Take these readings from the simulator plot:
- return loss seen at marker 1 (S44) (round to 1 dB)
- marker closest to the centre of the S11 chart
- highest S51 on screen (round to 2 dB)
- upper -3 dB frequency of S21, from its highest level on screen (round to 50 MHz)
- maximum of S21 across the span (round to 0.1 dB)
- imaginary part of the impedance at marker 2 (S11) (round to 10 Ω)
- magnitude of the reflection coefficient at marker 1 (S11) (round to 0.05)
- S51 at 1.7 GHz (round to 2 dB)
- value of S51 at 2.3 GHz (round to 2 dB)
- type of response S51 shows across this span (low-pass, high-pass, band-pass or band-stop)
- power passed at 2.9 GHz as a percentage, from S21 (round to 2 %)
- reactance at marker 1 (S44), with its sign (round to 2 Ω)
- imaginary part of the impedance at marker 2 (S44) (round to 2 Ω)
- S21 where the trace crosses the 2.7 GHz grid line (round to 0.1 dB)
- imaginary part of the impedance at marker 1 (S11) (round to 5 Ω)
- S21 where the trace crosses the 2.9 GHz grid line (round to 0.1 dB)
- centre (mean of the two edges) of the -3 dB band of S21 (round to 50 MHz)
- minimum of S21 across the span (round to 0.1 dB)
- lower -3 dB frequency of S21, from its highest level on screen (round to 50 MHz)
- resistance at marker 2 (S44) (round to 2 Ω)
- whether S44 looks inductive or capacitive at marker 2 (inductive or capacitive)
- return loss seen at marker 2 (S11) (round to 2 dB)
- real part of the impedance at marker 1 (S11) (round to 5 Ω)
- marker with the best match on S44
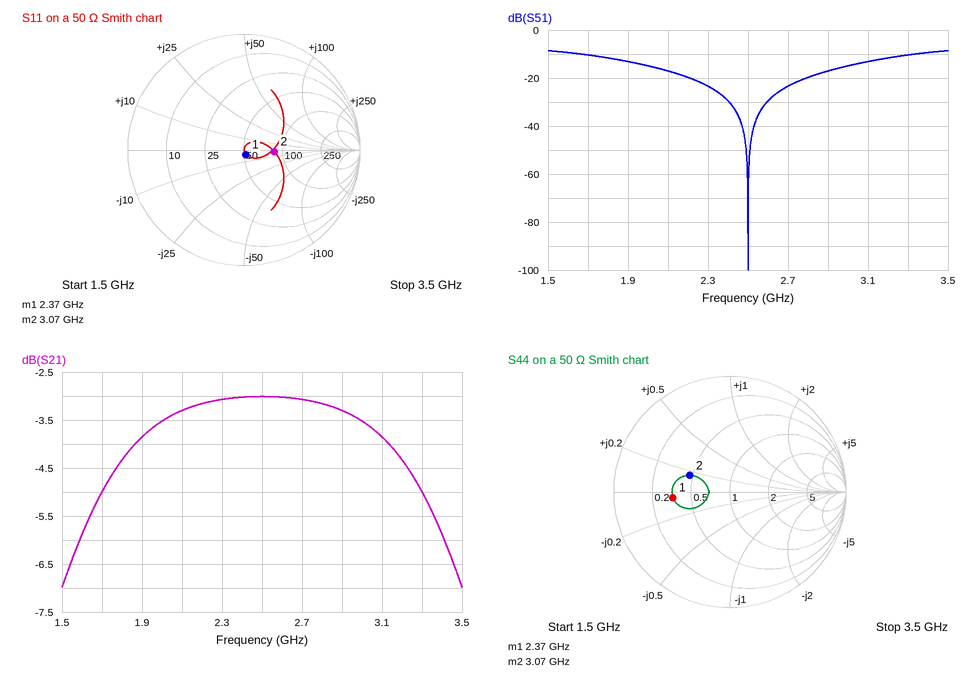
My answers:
6 dB
marker 1
-8 dB
3.40 GHz
-3.0 dB
0 Ω
0.05
-10 dB
-24 dB
band-stop
46 %
-2 Ω
+8 Ω
-3.1 dB
-5 Ω
-3.3 dB
2.50 GHz
-7.0 dB
1.60 GHz
24 Ω
inductive
12 dB
50 Ω
marker 2
